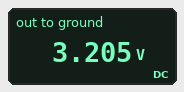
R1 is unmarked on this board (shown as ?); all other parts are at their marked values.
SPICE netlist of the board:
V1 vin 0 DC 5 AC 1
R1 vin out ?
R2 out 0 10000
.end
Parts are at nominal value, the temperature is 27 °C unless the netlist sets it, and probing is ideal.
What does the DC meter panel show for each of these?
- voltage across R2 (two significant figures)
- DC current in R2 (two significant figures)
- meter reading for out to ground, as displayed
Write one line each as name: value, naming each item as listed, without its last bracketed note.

voltage across R2: 3.2 V
DC current in R2: 320 µA
meter reading for out to ground, as displayed: 3.205 V
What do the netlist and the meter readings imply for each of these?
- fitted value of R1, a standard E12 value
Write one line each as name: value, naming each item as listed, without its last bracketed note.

fitted value of R1, a standard E12 value: 5.6 kΩ
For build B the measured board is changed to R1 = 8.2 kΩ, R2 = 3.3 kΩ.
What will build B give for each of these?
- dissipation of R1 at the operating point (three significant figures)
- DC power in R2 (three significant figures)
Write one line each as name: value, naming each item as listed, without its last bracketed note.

dissipation of R1 at the operating point: 1.55 mW
DC power in R2: 624 µW
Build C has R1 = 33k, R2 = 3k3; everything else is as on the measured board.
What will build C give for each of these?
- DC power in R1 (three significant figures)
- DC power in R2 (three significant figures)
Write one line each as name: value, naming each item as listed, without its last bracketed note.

DC power in R1: 626 µW
DC power in R2: 62.6 µW
